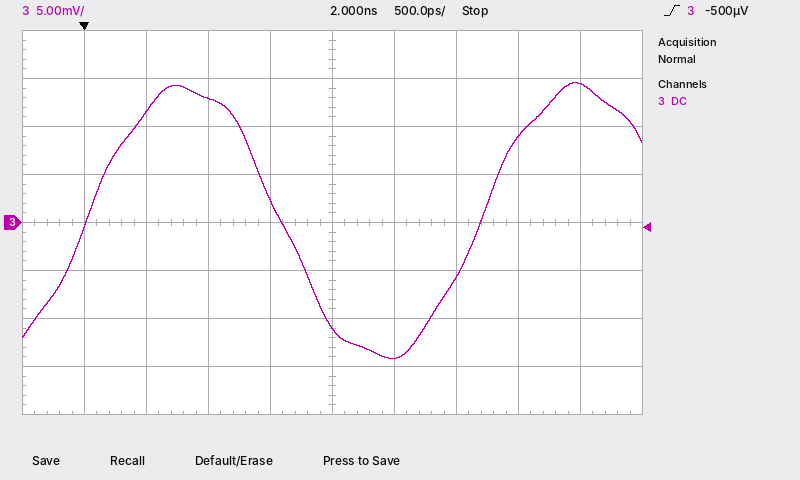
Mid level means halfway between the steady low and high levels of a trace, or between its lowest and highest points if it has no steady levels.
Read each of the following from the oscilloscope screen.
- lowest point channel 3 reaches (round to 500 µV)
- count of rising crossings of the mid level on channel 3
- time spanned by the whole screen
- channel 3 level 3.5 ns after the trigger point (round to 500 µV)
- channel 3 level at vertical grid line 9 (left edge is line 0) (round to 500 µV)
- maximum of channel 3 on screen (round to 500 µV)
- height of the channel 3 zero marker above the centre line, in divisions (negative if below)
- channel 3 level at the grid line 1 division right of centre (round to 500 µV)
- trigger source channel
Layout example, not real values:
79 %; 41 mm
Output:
-14.0 mV; 2; 5 ns; 9.0 mV; 14.5 mV; 14.5 mV; 0.0 div; -14.0 mV; channel 3
